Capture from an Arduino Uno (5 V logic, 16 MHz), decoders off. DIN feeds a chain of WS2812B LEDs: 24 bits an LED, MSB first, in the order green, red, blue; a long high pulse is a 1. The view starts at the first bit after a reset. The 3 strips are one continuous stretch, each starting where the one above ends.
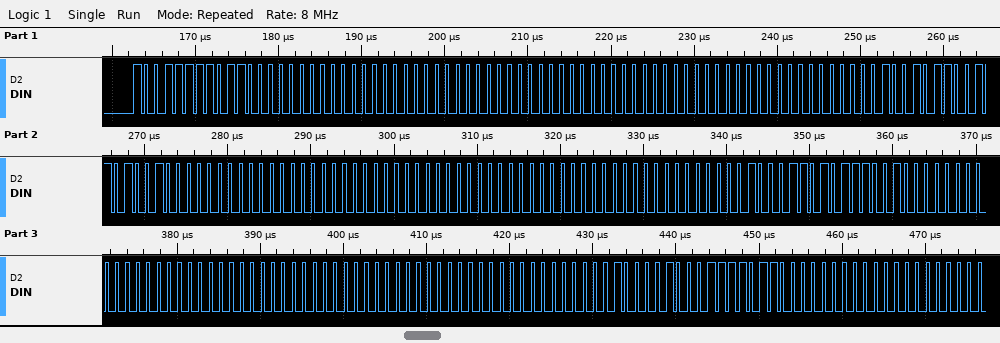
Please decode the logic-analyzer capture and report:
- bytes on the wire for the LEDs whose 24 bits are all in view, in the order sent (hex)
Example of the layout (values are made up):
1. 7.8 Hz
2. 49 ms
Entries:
1. 9F 60 00 00 00 00 00 00 00 96 69 00 00 00 00 00 00 00 8D 72 00 00 00 00 00 00 00 84 7B 00
